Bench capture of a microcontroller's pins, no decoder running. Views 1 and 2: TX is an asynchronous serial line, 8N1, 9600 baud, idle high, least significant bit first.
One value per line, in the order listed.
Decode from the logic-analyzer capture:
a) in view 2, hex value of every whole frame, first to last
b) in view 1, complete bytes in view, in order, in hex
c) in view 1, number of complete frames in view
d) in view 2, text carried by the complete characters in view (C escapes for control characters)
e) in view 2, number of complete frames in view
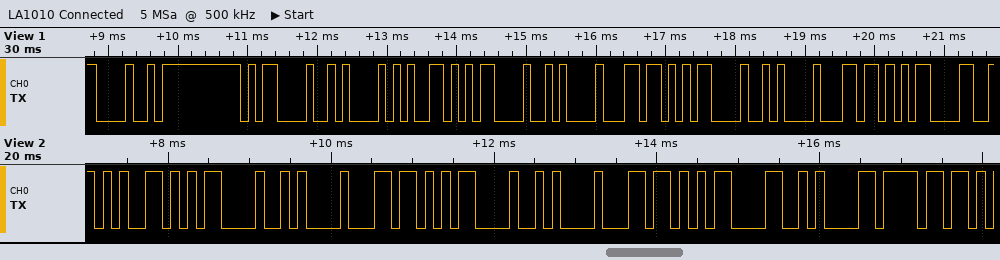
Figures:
0x65 0x0D 0x0A 0x6C 0x0D 0x0A 0x6C 0x0D 0x0A 0x6F
0x48 0x0D 0x0A 0x65 0x0D 0x0A 0x6C 0x0D 0x0A 0x6C 0x0D
11
"e\r\nl\r\nl\r\no"
10
